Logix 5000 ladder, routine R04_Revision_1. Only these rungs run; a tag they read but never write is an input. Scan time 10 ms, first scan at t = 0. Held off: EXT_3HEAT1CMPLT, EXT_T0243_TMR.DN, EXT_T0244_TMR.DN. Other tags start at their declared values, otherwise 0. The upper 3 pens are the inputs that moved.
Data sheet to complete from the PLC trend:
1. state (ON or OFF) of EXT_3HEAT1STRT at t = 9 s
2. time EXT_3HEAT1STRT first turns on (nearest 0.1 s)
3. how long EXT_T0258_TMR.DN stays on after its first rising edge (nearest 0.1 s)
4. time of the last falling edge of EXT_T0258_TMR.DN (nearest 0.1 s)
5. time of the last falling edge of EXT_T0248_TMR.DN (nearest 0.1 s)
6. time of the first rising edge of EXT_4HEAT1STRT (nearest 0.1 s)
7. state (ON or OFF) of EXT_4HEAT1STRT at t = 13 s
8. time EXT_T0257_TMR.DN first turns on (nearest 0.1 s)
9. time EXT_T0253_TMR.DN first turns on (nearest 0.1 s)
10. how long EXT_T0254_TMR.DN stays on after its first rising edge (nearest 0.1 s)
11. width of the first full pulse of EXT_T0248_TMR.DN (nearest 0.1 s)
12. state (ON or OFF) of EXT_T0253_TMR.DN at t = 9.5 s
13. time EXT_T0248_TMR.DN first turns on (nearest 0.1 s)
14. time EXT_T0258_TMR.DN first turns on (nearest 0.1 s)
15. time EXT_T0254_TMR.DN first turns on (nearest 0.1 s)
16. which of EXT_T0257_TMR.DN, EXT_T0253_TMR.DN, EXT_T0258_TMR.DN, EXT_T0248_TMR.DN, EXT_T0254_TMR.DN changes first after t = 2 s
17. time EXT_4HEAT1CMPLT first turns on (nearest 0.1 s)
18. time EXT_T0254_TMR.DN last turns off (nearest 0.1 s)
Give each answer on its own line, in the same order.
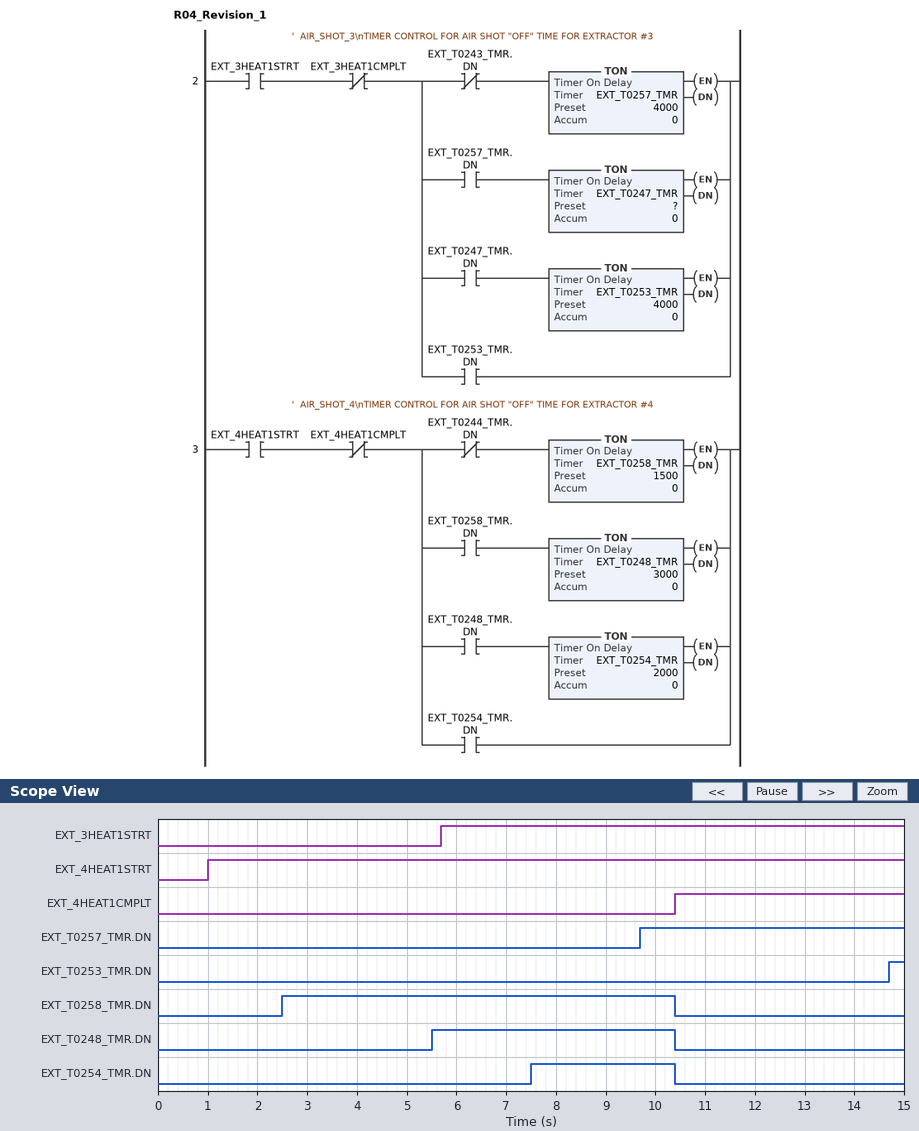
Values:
ON
5.7 s
7.9 s
10.4 s
10.4 s
1.0 s
ON
9.7 s
14.7 s
2.9 s
4.9 s
OFF
5.5 s
2.5 s
7.5 s
EXT_T0258_TMR.DN
10.4 s
10.4 s
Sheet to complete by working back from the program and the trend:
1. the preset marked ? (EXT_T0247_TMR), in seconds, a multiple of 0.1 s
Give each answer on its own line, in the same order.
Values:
1.0 s
